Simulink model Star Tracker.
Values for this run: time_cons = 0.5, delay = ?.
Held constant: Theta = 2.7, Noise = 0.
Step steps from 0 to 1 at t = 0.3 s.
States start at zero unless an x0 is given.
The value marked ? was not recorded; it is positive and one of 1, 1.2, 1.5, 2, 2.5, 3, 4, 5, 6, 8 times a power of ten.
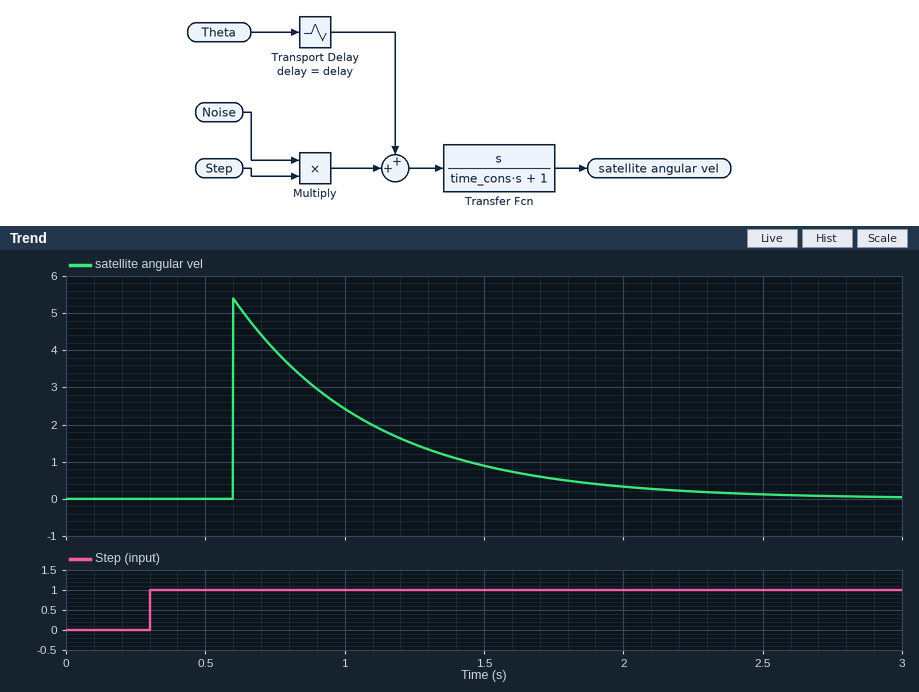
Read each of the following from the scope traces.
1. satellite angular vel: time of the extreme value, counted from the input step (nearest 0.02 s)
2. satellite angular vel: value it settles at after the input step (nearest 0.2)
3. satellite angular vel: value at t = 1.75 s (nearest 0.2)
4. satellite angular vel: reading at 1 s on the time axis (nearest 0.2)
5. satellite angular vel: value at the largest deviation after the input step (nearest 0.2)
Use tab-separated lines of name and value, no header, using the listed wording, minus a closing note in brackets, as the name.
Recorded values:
satellite angular vel: time of the extreme value, counted from the input step	0.30 s
satellite angular vel: value it settles at after the input step	0.0
satellite angular vel: value at t = 1.75 s	0.6
satellite angular vel: reading at 1 s on the time axis	2.4
satellite angular vel: value at the largest deviation after the input step	5.4
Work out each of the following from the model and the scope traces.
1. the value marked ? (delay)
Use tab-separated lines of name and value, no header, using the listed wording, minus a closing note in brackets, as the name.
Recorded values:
the value marked ?	0.6
